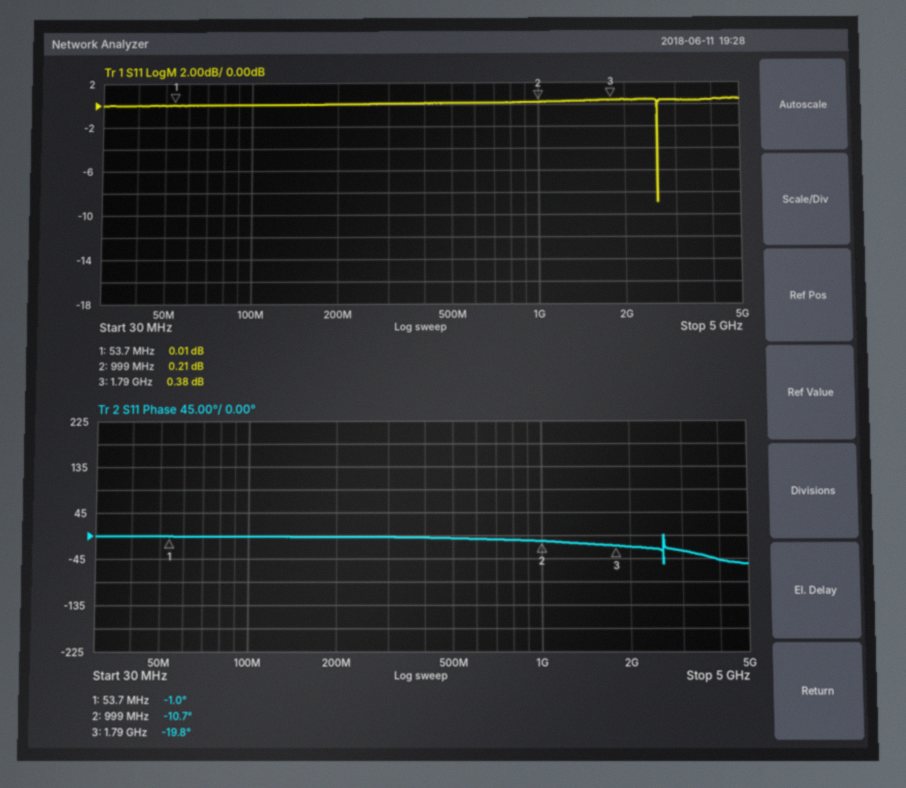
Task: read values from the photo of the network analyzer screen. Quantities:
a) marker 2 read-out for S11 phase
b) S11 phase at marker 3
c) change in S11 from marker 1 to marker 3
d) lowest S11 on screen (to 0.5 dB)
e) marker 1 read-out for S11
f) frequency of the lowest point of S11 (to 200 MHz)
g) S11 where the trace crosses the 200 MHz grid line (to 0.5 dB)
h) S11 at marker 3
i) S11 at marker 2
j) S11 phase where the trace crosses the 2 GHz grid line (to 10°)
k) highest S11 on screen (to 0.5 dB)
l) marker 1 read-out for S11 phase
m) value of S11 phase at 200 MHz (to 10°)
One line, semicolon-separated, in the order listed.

-10.7°; -19.8°; 0.37 dB; -9.0 dB; 0.01 dB; 2.6 GHz; 0.0 dB; 0.38 dB; 0.21 dB; -20°; 0.5 dB; -1.0°; 0°
